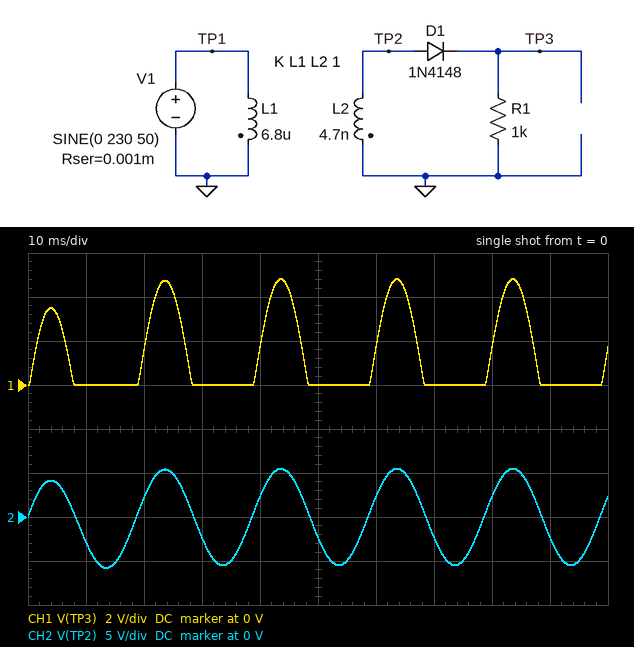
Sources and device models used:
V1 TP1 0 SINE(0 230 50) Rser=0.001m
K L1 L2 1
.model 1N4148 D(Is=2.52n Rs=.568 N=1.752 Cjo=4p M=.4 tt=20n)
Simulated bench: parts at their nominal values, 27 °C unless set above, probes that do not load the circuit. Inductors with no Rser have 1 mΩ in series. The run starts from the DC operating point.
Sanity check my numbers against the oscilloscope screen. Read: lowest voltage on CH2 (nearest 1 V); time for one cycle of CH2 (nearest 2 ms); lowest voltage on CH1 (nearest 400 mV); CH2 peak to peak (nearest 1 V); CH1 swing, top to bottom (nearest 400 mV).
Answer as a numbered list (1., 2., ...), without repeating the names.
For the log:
1. -6 V
2. 20 ms
3. 0 V
4. 11 V
5. 4.8 V
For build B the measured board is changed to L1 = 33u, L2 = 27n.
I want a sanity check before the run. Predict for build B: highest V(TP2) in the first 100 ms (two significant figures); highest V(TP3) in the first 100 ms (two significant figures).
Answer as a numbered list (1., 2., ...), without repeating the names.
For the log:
1. 6.5 V
2. 5.8 V
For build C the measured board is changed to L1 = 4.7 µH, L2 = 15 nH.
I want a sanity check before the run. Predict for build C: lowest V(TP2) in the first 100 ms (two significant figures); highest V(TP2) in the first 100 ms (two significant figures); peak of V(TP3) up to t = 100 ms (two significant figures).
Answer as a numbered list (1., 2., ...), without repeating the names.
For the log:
1. -11 V
2. 11 V
3. 10 V
